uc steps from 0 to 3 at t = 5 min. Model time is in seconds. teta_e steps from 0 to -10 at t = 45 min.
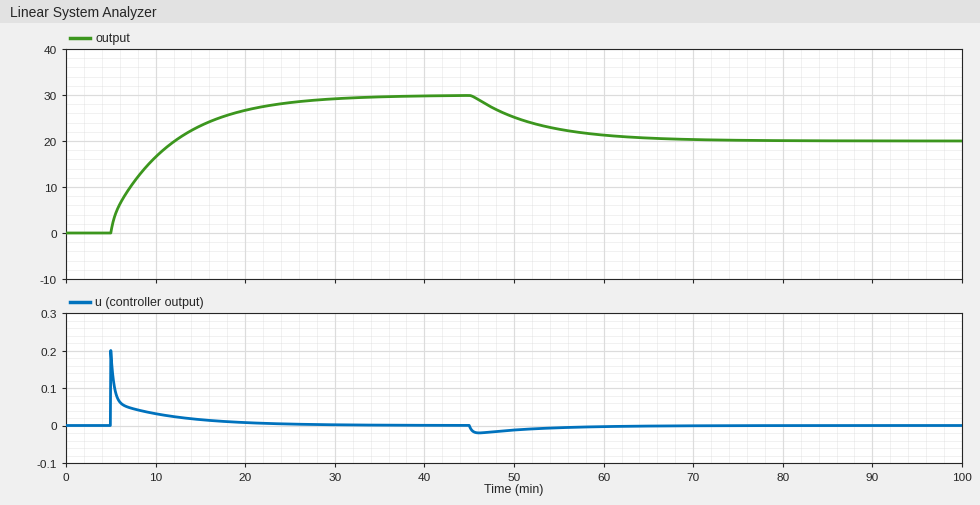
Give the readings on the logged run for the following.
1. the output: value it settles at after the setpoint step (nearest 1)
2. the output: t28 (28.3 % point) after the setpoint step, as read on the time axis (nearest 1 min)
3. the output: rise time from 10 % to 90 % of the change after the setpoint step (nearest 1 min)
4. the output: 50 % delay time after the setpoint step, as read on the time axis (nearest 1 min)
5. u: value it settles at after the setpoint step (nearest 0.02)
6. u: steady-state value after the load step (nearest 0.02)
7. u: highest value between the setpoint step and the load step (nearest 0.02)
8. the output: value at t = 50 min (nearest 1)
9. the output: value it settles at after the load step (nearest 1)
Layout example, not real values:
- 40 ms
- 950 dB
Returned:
- 30
- 7 min
- 15 min
- 9 min
- 0.00
- 0.00
- 0.20
- 25
- 20
